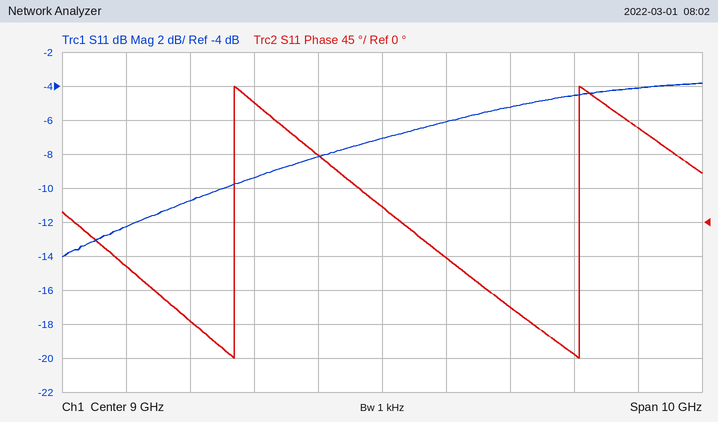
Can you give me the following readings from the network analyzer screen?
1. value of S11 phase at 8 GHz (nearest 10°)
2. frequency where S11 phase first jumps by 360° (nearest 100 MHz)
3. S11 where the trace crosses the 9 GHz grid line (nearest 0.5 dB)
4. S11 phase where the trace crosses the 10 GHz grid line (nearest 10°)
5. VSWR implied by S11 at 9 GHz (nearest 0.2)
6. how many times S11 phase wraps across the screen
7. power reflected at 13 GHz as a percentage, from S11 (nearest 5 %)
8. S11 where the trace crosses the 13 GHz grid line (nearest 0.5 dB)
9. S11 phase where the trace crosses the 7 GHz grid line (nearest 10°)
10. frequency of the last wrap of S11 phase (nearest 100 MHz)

90°
6.7 GHz
-7.0 dB
-50°
2.6
2
40 %
-4.0 dB
160°
12.1 GHz
